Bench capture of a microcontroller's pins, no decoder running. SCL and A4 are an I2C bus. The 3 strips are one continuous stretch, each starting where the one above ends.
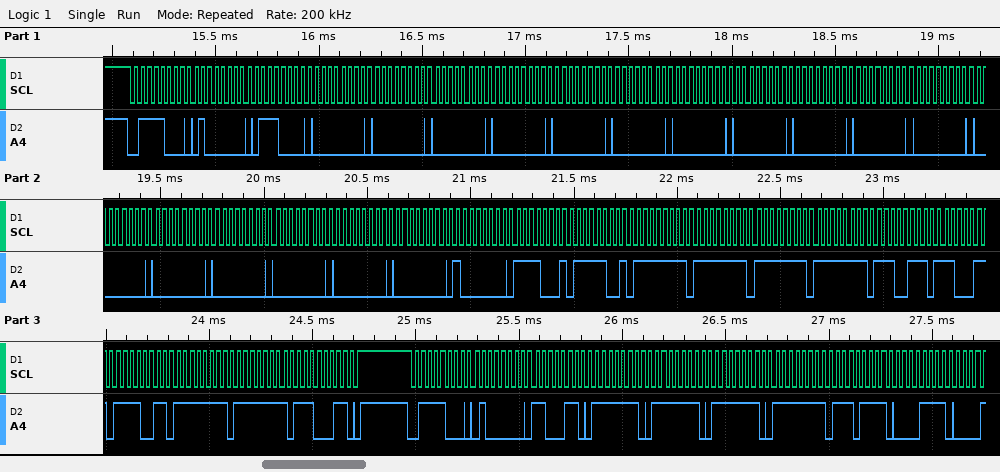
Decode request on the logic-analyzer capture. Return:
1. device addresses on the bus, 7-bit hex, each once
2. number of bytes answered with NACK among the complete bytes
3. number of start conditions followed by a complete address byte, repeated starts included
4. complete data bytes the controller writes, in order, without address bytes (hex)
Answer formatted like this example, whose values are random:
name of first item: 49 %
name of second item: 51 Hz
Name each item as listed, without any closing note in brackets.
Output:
device addresses on the bus, 7-bit hex, each once: 0x3C
number of bytes answered with NACK among the complete bytes: 0
number of start conditions followed by a complete address byte, repeated starts included: 2
complete data bytes the controller writes, in order, without address bytes: 40 70 00 00 00 00 00 00 00 00 00 00 00 00 00 00 00 00 00 80 F1 F9 FF FF FF FF E7 E3 F3 FF FF E3 40 C6 FE FE FE FF EF 0F
